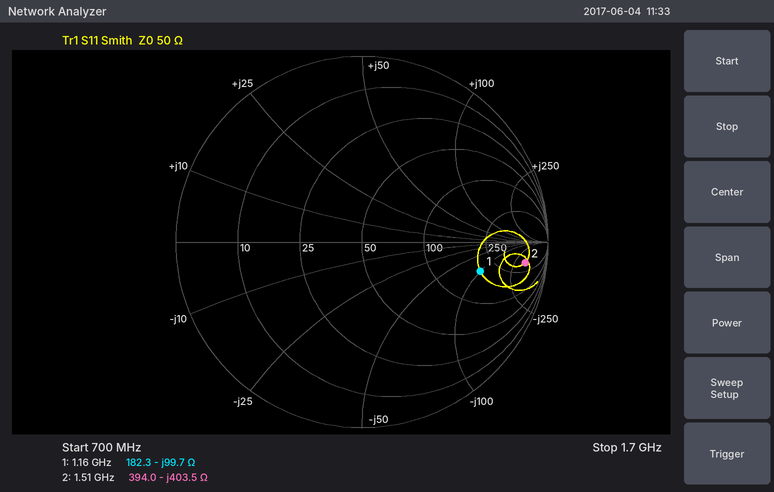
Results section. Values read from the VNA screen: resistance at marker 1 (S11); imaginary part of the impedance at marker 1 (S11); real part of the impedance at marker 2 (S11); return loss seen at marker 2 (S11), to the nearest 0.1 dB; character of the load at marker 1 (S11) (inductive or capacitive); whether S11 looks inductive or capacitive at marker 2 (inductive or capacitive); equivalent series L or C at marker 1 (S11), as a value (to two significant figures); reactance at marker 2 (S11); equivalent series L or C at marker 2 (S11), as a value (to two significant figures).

182.3 Ω
-99.7 Ω
394.0 Ω
1.1 dB
capacitive
capacitive
1.4 pF
-403.5 Ω
260 fF
